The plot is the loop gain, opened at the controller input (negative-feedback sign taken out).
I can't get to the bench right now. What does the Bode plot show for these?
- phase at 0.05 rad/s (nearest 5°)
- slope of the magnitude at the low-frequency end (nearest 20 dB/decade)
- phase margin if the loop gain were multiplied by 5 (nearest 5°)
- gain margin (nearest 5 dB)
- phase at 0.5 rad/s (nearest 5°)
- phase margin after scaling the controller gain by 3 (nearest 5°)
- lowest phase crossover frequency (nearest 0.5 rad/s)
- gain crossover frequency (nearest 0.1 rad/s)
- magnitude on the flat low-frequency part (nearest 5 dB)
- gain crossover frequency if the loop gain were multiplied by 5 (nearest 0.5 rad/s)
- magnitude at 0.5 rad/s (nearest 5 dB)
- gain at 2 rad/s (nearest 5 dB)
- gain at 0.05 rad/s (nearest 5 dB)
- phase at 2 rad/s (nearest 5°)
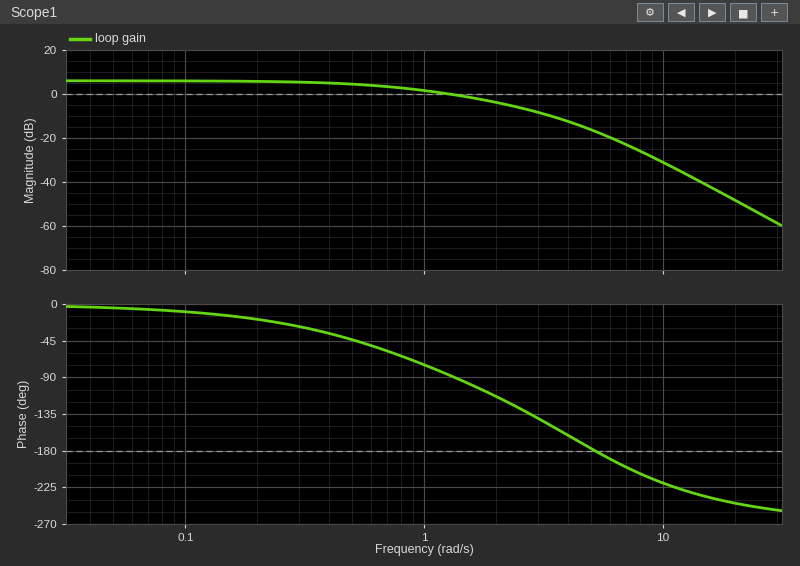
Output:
-5°
0 dB/decade
10°
15 dB
-45°
35°
5.0 rad/s
1.3 rad/s
5 dB
4.5 rad/s
5 dB
-5 dB
5 dB
-115°
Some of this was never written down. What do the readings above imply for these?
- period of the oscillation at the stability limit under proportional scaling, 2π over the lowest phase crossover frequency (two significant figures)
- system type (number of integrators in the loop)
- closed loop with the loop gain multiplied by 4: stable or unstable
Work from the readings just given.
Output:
1.3 s
0
stable
